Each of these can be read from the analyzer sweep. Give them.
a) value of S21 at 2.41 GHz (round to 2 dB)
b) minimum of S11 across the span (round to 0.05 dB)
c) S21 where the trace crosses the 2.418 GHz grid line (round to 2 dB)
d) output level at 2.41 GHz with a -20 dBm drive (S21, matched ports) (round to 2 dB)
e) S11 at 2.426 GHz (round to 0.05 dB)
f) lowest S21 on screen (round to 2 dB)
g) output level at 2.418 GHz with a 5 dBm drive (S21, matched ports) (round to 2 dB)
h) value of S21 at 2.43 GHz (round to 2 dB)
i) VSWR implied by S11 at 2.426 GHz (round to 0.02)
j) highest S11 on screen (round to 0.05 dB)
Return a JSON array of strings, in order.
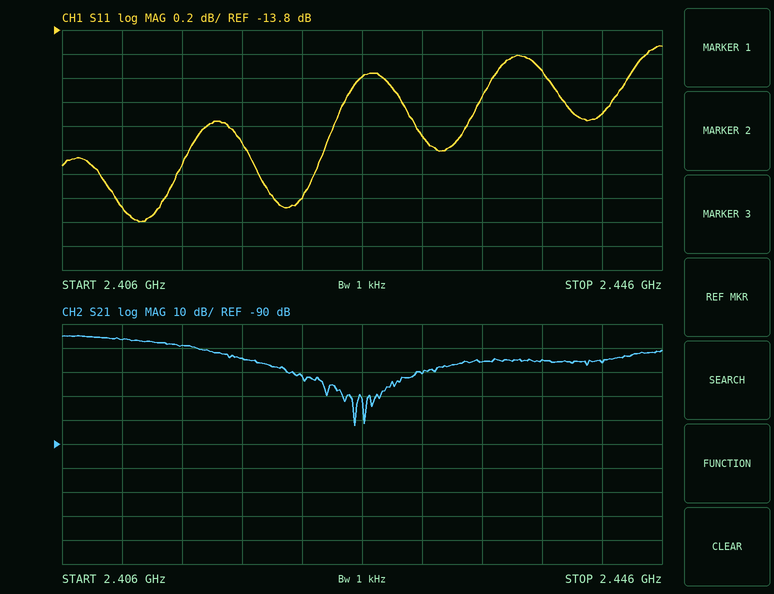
["-46 dB", "-15.40 dB", "-54 dB", "-66 dBm", "-14.20 dB", "-82 dB", "-50 dBm", "-60 dB", "1.48", "-13.95 dB"]
